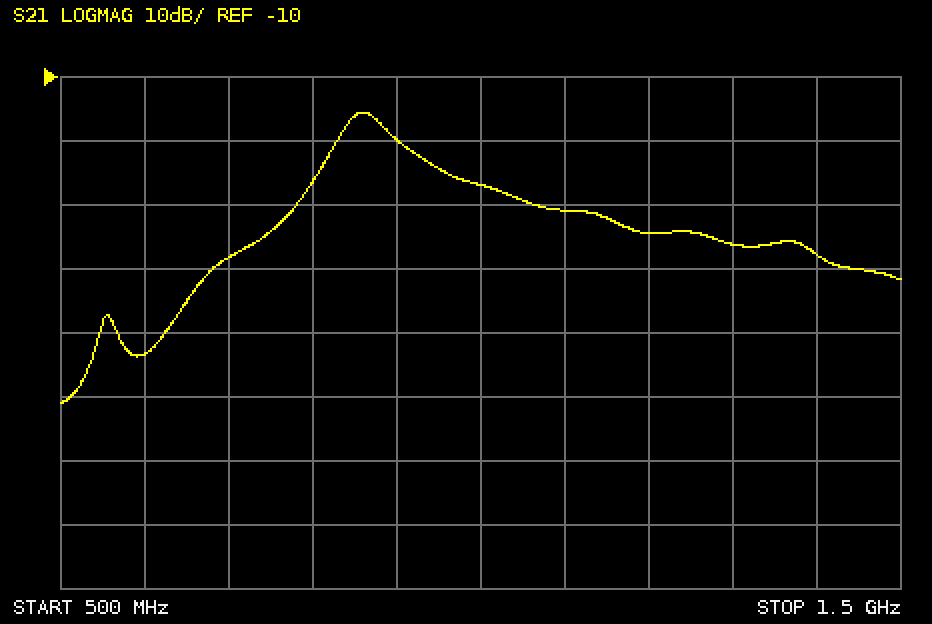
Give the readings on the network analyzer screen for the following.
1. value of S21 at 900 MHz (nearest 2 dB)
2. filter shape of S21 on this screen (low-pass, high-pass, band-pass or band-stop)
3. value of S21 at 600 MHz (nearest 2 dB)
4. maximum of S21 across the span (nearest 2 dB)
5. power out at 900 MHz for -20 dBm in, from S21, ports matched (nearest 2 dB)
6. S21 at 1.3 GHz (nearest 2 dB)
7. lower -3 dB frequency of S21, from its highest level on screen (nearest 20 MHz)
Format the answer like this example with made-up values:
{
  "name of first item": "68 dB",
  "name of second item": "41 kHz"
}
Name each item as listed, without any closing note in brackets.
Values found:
{
  "value of S21 at 900 MHz": "-20 dB",
  "filter shape of S21 on this screen": "band-pass",
  "value of S21 at 600 MHz": "-54 dB",
  "maximum of S21 across the span": "-16 dB",
  "power out at 900 MHz for -20 dBm in, from S21, ports matched": "-40 dBm",
  "S21 at 1.3 GHz": "-36 dB",
  "lower -3 dB frequency of S21, from its highest level on screen": "840 MHz"
}
